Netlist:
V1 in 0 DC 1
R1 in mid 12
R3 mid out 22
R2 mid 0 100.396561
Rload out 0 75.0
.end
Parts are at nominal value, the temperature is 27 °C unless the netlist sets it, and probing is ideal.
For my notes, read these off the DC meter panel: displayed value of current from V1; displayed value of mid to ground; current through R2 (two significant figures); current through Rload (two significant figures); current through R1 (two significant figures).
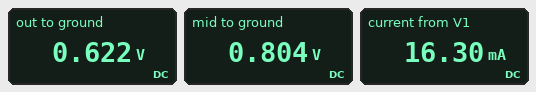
16.30 mA
0.804 V
8.0 mA
8.3 mA
16 mA
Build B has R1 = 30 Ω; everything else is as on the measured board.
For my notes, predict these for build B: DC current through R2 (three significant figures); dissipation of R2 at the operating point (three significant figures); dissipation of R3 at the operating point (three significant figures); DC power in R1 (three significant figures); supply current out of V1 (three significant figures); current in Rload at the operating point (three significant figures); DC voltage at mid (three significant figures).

6.19 mA
3.85 mW
904 µW
4.77 mW
12.6 mA
6.41 mA
622 mV
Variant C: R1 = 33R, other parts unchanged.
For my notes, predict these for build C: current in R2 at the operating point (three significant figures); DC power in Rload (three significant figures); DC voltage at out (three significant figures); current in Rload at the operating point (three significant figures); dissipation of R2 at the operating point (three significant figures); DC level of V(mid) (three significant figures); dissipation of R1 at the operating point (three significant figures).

5.97 mA
2.86 mW
463 mV
6.18 mA
3.58 mW
599 mV
4.87 mW
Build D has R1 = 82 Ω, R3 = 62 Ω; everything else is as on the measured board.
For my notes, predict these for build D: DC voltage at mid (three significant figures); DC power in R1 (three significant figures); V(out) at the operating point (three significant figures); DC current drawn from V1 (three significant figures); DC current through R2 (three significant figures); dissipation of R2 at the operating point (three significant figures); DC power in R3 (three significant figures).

414 mV
4.19 mW
227 mV
7.15 mA
4.12 mA
1.71 mW
566 µW
